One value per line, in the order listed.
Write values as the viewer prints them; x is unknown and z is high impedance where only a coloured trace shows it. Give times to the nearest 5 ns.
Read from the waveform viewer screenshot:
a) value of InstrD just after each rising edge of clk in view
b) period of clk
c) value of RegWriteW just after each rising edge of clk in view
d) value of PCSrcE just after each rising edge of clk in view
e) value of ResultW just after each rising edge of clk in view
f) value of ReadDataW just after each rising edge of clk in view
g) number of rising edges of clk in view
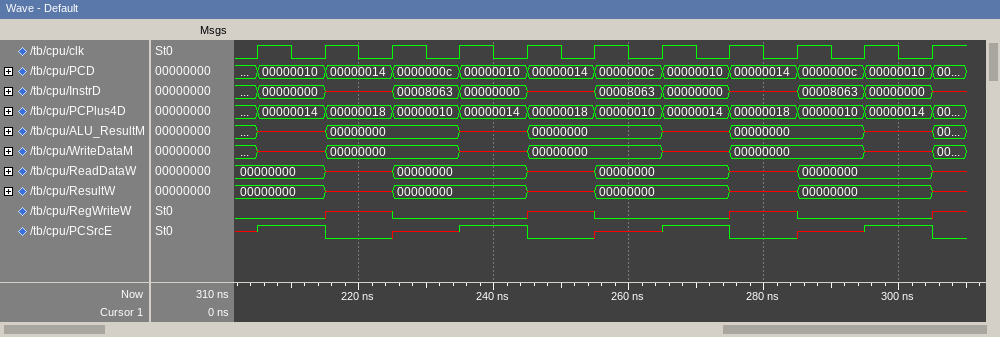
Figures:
00000000, x, 00008063, 00000000, x, 00008063, 00000000, x, 00008063, 00000000, x
10 ns
0 x 0 0 x 0 0 x 0 0 x
1 0 x 1 0 x 1 0 x 1 0
00000000, x, 00000000, 00000000, x, 00000000, 00000000, x, 00000000, 00000000, x
00000000, x, 00000000, 00000000, x, 00000000, 00000000, x, 00000000, 00000000, x
11
